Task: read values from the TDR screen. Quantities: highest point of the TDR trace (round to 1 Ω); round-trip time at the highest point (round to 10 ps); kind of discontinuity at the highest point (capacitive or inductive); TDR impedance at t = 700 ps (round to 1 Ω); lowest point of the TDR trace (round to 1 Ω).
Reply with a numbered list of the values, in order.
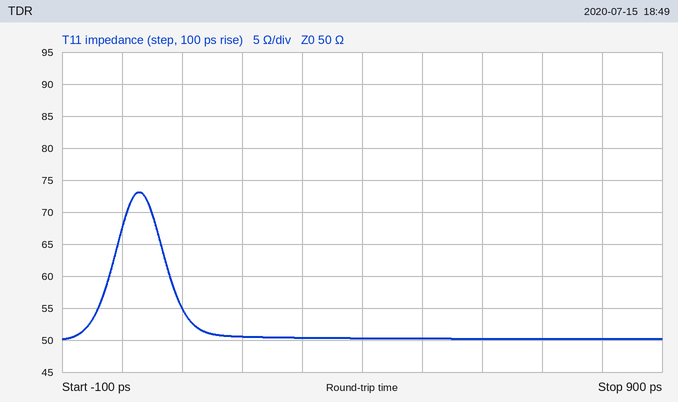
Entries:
1. 73 Ω
2. 30 ps
3. inductive
4. 50 Ω
5. 50 Ω
